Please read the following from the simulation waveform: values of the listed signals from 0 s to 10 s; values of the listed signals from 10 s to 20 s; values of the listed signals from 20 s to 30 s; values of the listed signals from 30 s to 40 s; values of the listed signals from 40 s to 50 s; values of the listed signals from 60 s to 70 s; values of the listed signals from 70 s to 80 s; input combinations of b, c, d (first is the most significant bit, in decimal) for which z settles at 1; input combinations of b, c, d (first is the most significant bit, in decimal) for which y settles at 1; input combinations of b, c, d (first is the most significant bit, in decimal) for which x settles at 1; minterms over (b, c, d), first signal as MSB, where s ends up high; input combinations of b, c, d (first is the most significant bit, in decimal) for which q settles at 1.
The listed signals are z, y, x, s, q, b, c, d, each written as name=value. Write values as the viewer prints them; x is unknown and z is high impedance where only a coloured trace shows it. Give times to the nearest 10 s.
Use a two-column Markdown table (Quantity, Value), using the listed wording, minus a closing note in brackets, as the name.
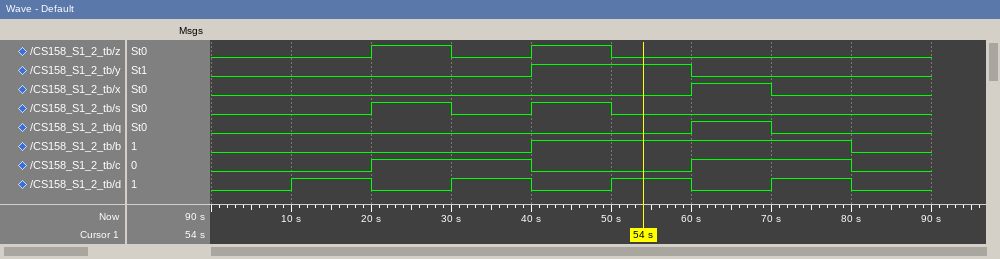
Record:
| Quantity | Value |
|---|---|
| values of the listed signals from 0 s to 10 s | z=0, y=0, x=0, s=0, q=0, b=0, c=0, d=0 |
| values of the listed signals from 10 s to 20 s | z=0, y=0, x=0, s=0, q=0, b=0, c=0, d=1 |
| values of the listed signals from 20 s to 30 s | z=1, y=0, x=0, s=1, q=0, b=0, c=1, d=0 |
| values of the listed signals from 30 s to 40 s | z=0, y=0, x=0, s=0, q=0, b=0, c=1, d=1 |
| values of the listed signals from 40 s to 50 s | z=1, y=1, x=0, s=1, q=0, b=1, c=0, d=0 |
| values of the listed signals from 60 s to 70 s | z=0, y=0, x=1, s=0, q=1, b=1, c=1, d=0 |
| values of the listed signals from 70 s to 80 s | z=0, y=0, x=0, s=0, q=0, b=1, c=1, d=1 |
| input combinations of b, c, d (first is the most significant bit, in decimal) for which z settles at 1 | 2, 4 |
| input combinations of b, c, d (first is the most significant bit, in decimal) for which y settles at 1 | 4, 5 |
| input combinations of b, c, d (first is the most significant bit, in decimal) for which x settles at 1 | 6 |
| minterms over (b, c, d), first signal as MSB, where s ends up high | 2, 4 |
| input combinations of b, c, d (first is the most significant bit, in decimal) for which q settles at 1 | 6 |
